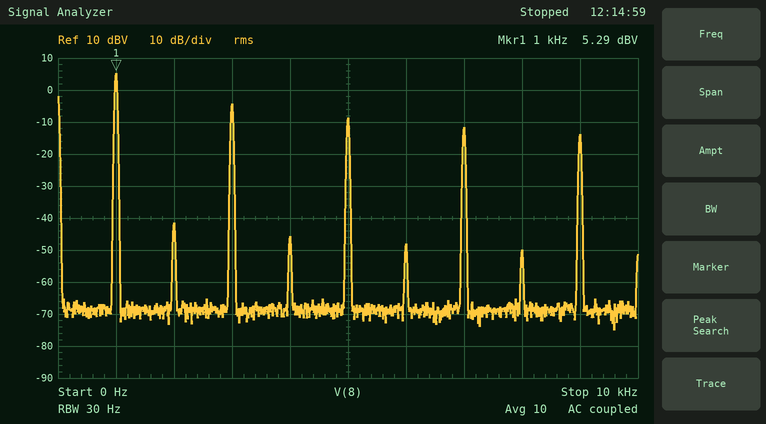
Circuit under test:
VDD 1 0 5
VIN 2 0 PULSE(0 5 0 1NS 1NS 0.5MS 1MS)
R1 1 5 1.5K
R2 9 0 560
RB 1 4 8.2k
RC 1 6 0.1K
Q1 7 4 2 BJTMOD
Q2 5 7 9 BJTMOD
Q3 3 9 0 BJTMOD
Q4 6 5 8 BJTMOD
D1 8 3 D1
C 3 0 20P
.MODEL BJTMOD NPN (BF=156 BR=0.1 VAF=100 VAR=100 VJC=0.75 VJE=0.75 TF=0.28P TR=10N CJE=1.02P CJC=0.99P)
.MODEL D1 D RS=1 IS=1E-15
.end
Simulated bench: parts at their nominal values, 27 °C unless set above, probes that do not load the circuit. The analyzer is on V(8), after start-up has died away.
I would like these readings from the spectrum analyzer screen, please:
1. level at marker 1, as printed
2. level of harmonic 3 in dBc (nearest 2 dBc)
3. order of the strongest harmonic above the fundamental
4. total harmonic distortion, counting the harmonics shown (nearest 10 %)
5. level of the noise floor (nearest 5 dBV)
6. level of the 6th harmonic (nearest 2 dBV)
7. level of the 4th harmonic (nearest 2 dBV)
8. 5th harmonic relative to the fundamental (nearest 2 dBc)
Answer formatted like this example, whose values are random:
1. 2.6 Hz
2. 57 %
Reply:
1. 5.29 dBV
2. -10 dBc
3. 3
4. 40 %
5. -70 dBV
6. -48 dBV
7. -46 dBV
8. -14 dBc
